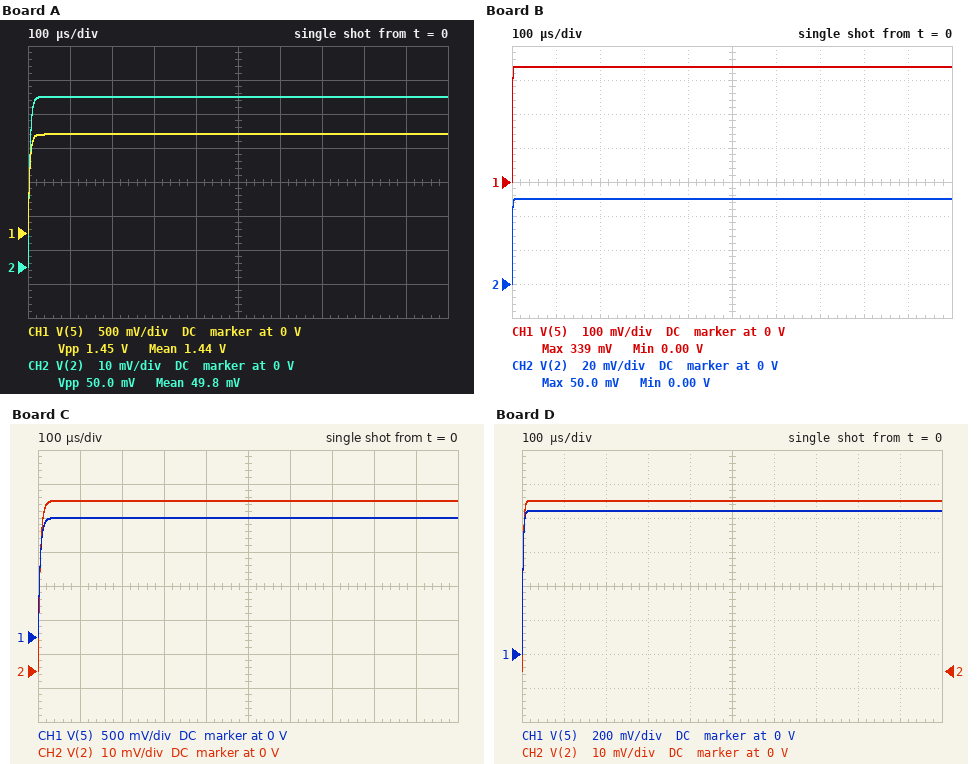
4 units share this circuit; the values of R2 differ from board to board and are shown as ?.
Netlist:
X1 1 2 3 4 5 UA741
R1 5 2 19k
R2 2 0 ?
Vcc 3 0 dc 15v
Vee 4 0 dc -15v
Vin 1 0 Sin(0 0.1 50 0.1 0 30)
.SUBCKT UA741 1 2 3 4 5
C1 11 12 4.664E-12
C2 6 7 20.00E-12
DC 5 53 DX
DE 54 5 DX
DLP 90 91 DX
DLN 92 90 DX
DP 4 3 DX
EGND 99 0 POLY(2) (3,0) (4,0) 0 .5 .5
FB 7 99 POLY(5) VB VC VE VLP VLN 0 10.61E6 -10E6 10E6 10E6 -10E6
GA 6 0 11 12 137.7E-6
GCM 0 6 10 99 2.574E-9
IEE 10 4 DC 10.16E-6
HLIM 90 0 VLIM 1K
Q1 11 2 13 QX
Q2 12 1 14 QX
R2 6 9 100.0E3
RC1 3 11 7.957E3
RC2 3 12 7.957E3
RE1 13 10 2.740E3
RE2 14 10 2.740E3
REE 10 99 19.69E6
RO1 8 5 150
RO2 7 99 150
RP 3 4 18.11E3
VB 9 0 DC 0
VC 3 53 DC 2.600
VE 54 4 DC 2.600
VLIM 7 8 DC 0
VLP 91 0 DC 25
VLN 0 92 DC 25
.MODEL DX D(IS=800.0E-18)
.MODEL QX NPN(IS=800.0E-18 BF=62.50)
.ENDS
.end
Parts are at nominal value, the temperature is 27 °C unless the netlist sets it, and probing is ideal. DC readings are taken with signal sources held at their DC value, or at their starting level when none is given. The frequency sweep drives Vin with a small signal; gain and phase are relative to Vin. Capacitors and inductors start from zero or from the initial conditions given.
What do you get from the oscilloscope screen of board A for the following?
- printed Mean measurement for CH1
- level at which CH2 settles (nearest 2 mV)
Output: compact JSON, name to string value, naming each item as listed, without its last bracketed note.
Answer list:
{"printed Mean measurement for CH1": "1.44 V", "level at which CH2 settles": "50 mV"}
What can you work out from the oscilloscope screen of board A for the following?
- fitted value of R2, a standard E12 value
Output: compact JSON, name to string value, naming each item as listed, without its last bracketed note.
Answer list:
{"fitted value of R2, a standard E12 value": "680 Ω"}
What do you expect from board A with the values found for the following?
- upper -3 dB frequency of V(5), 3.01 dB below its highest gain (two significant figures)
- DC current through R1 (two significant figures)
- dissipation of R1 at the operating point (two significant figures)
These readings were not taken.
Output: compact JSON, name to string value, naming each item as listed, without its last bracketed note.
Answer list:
{"upper -3 dB frequency of V(5), 3.01 dB below its highest gain": "38 kHz", "DC current through R1": "74 µA", "dissipation of R1 at the operating point": "100 µW"}
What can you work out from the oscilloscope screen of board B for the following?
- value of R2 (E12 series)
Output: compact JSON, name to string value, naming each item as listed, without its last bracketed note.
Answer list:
{"value of R2": "3.3 kΩ"}
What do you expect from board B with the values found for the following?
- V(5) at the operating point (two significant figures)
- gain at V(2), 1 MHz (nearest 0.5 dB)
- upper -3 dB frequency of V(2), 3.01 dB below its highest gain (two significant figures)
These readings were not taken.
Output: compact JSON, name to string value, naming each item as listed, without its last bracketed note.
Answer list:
{"V(5) at the operating point": "340 mV", "gain at V(2), 1 MHz": "-16.5 dB", "upper -3 dB frequency of V(2), 3.01 dB below its highest gain": "170 kHz"}
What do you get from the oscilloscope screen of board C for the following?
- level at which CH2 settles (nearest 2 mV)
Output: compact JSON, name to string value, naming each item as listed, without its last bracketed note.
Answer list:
{"level at which CH2 settles": "50 mV"}
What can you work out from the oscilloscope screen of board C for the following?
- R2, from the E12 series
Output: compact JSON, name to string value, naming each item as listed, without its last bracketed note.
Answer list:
{"R2, from the E12 series": "560 Ω"}
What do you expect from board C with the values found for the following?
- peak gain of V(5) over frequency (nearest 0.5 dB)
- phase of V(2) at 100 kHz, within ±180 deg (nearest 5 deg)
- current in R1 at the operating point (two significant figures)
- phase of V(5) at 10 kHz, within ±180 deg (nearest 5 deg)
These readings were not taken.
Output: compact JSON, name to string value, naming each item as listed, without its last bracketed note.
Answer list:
{"peak gain of V(5) over frequency": "31.0 dB", "phase of V(2) at 100 kHz, within ±180 deg": "-75 deg", "current in R1 at the operating point": "89 µA", "phase of V(5) at 10 kHz, within ±180 deg": "-20 deg"}
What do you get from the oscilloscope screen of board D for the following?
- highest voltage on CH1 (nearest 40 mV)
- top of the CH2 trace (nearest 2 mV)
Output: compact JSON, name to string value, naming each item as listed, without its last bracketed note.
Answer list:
{"highest voltage on CH1": "840 mV", "top of the CH2 trace": "50 mV"}
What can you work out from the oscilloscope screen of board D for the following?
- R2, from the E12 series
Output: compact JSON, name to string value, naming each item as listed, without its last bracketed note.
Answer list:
{"R2, from the E12 series": "1.2 kΩ"}
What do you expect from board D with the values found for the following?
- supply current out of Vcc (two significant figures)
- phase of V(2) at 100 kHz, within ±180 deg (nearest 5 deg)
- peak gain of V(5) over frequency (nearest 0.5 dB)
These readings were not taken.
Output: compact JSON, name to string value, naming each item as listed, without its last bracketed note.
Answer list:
{"supply current out of Vcc": "1.7 mA", "phase of V(2) at 100 kHz, within ±180 deg": "-60 deg", "peak gain of V(5) over frequency": "24.5 dB"}
